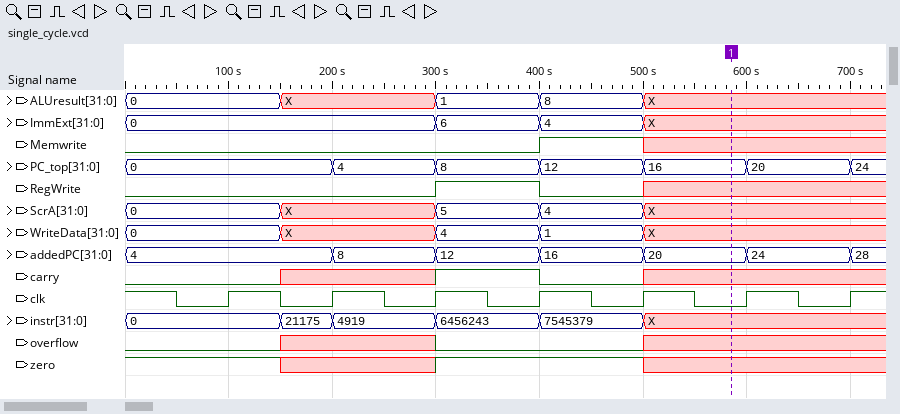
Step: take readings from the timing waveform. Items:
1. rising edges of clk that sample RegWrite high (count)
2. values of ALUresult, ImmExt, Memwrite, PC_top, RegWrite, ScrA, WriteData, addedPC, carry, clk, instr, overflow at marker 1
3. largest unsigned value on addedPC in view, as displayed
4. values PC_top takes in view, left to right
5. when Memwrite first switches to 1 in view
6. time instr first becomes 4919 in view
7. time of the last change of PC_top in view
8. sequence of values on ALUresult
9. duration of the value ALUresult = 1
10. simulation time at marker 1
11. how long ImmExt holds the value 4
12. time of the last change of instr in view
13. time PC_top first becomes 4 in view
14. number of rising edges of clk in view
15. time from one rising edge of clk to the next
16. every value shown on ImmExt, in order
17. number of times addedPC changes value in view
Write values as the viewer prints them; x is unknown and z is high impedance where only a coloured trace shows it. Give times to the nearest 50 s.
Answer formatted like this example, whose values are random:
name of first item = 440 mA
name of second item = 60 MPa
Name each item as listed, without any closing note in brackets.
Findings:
rising edges of clk that sample RegWrite high = 1
values of ALUresult, ImmExt, Memwrite, PC_top, RegWrite, ScrA, WriteData, addedPC, carry, clk, instr, overflow at marker 1 = ALUresult=X, ImmExt=X, Memwrite=x, PC_top=16, RegWrite=x, ScrA=X, WriteData=X, addedPC=20, carry=x, clk=0, instr=X, overflow=x
largest unsigned value on addedPC in view, as displayed = 28
values PC_top takes in view, left to right = 0, 4, 8, 12, 16, 20, 24
when Memwrite first switches to 1 in view = 400 s
time instr first becomes 4919 in view = 200 s
time of the last change of PC_top in view = 700 s
sequence of values on ALUresult = 0, X, 1, 8, X
duration of the value ALUresult = 1 = 100 s
simulation time at marker 1 = 600 s
how long ImmExt holds the value 4 = 100 s
time of the last change of instr in view = 500 s
time PC_top first becomes 4 in view = 200 s
number of rising edges of clk in view = 7
time from one rising edge of clk to the next = 100 s
every value shown on ImmExt, in order = 0, 6, 4, X
number of times addedPC changes value in view = 6
